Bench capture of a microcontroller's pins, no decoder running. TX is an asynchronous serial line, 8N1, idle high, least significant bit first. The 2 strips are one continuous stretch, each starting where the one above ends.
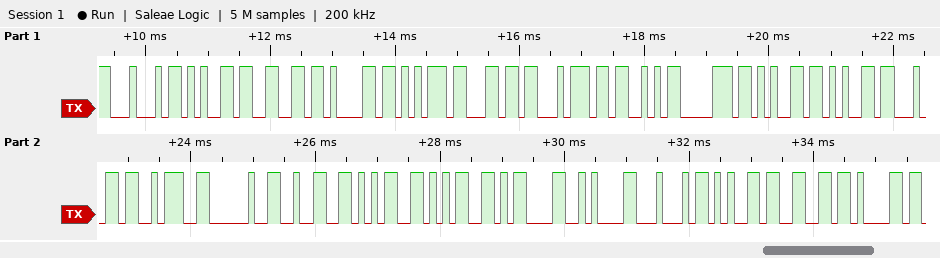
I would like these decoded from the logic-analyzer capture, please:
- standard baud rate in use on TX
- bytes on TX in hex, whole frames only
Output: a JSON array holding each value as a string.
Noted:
["9600 baud", "44 65 66 61 75 6C 74 53 70 65 65 64 3A 20 32 35 35 0D 0A 44 65 66 61"]
